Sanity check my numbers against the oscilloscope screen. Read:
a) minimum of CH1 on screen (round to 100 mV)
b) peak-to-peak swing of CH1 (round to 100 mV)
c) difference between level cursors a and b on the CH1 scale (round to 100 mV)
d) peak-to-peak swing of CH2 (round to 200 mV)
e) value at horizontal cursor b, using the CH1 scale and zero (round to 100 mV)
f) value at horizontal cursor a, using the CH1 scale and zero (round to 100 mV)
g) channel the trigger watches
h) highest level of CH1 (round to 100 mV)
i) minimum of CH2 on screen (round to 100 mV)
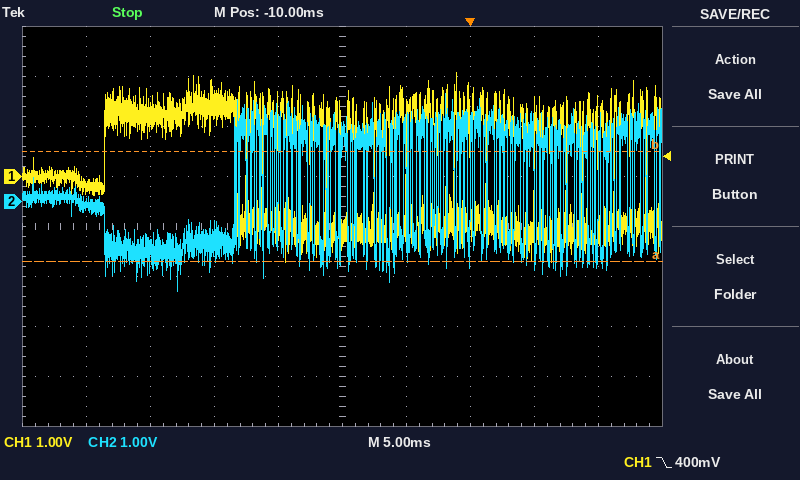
-1.7 V
3.8 V
2.2 V
4.0 V
500 mV
-1.7 V
CH1
2.1 V
-1.8 V
